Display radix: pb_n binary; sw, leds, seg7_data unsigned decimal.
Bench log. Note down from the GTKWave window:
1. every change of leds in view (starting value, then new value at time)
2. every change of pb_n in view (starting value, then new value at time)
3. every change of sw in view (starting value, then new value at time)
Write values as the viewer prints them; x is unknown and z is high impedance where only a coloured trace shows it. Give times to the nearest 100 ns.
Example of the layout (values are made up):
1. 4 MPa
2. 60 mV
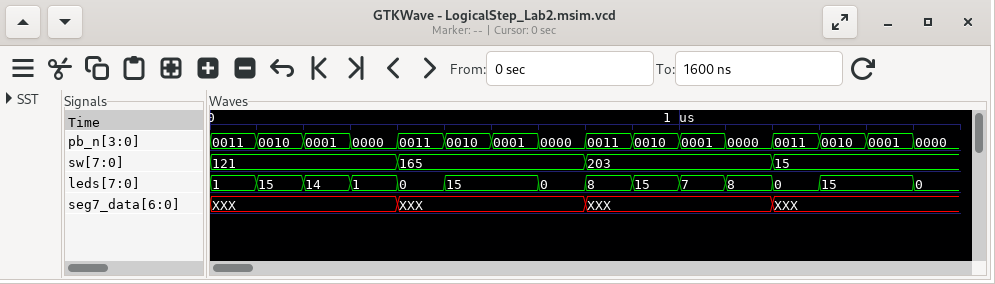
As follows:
1. 1, 15 at 100 ns, 14 at 200 ns, 1 at 300 ns, 0 at 400 ns, 15 at 500 ns, 0 at 700 ns, 8 at 800 ns, 15 at 900 ns, 7 at 1000 ns, 8 at 1100 ns, 0 at 1200 ns, 15 at 1300 ns, 0 at 1500 ns
2. 0011, 0010 at 100 ns, 0001 at 200 ns, 0000 at 300 ns, 0011 at 400 ns, 0010 at 500 ns, 0001 at 600 ns, 0000 at 700 ns, 0011 at 800 ns, 0010 at 900 ns, 0001 at 1000 ns, 0000 at 1100 ns, 0011 at 1200 ns, 0010 at 1300 ns, 0001 at 1400 ns, 0000 at 1500 ns
3. 121, 165 at 400 ns, 203 at 800 ns, 15 at 1200 ns
